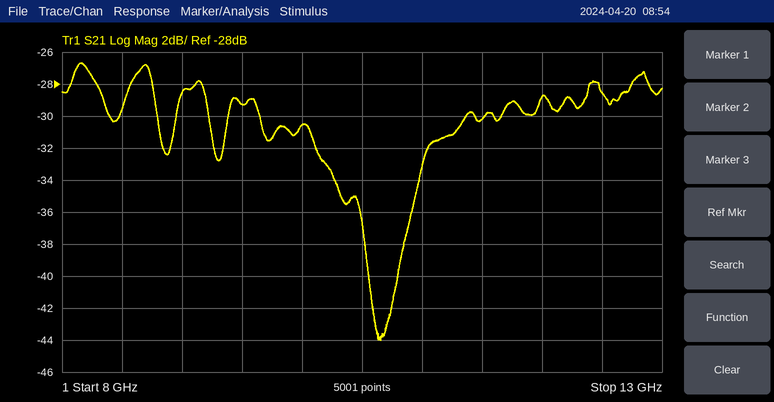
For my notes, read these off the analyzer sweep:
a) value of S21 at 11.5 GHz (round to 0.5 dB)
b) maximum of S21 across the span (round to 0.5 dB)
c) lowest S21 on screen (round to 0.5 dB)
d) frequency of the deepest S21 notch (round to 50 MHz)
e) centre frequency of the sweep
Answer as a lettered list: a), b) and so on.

a) -30.0 dB
b) -26.5 dB
c) -44.0 dB
d) 10.65 GHz
e) 10.5 GHz
